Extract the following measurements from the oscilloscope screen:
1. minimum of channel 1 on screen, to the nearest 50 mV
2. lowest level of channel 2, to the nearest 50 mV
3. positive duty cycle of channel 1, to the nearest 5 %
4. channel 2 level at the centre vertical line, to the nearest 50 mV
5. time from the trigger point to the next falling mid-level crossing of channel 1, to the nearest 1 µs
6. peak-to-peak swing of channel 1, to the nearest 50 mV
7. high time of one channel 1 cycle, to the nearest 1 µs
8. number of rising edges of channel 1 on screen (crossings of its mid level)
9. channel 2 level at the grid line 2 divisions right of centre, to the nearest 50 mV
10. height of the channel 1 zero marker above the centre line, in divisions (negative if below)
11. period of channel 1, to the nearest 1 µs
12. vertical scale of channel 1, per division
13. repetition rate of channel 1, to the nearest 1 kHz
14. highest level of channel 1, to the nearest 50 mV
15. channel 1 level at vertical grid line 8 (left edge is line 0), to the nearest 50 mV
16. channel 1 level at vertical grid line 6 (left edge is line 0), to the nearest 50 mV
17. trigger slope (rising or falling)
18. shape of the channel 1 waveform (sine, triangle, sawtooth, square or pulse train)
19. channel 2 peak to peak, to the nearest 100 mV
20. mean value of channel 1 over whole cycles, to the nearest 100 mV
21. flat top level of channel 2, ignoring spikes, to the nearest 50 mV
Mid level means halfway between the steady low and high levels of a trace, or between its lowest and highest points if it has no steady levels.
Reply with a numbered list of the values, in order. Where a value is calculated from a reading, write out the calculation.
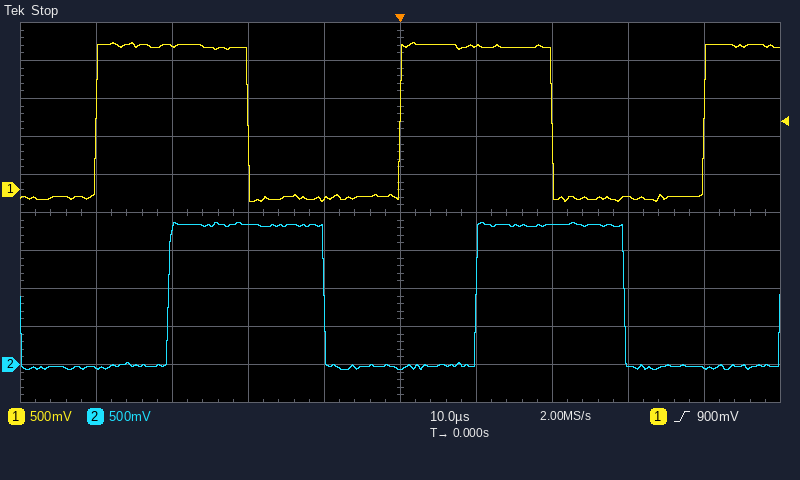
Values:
1. -150 mV
2. -50 mV
3. 20 µs / 40 µs ≈ 50 %
4. -50 mV
5. 20 µs
6. 1.95 V − (-150 mV) = 2.10 V
7. 20 µs
8. 3
9. 1.85 V
10. +0.6 div
11. 40 µs
12. 500 mV
13. 1 / 40 µs ≈ 25 kHz
14. 1.95 V
15. -100 mV
16. 1.90 V
17. rising
18. square
19. 1.90 V
20. -150 mV + 0.5 × (1.95 V − (-150 mV)) ≈ 900 mV
21. 1.85 V
